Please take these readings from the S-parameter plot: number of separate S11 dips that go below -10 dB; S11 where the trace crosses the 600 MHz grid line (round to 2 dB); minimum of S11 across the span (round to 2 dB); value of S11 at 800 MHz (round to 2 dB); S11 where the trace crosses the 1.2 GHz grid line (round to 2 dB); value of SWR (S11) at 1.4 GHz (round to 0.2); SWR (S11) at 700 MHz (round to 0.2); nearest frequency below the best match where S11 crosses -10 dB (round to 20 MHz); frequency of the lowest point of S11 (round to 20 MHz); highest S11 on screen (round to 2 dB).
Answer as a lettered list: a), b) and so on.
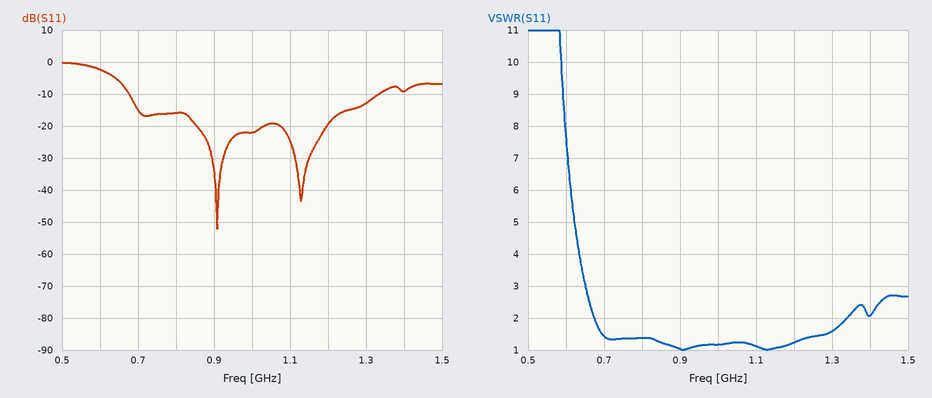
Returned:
a) 2
b) -2 dB
c) -52 dB
d) -16 dB
e) -20 dB
f) 2.0
g) 1.4
h) 680 MHz
i) 900 MHz
j) 0 dB
